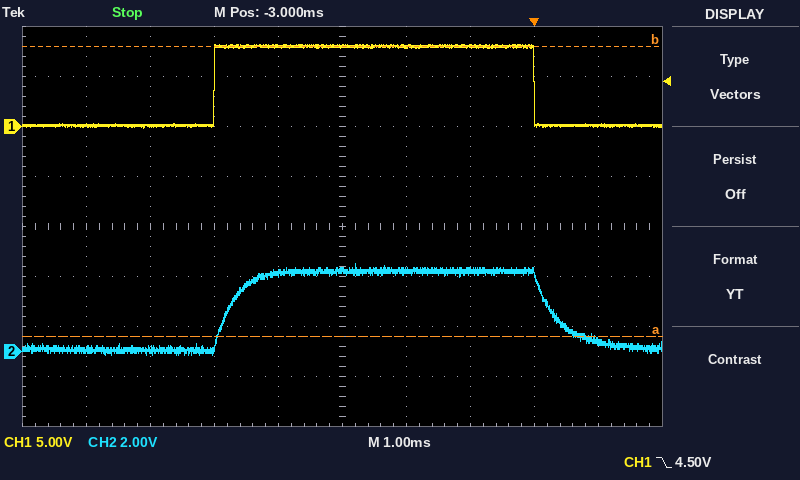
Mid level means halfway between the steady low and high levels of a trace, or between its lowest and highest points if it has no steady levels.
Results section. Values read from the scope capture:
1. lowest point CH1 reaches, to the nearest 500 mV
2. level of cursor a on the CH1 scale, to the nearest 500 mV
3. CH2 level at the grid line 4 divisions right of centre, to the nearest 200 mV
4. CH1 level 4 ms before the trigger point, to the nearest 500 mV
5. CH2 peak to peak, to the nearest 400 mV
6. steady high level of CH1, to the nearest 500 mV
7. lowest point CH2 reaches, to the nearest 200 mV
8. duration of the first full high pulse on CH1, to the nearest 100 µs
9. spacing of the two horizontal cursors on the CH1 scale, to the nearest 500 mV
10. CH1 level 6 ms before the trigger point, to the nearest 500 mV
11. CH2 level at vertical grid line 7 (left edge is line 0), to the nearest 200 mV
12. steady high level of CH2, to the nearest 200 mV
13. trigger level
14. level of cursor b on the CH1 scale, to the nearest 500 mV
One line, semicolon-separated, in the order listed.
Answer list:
0.0 V; -21.0 V; 400 mV; 8.0 V; 3.6 V; 8.0 V; -200 mV; 5.0 ms; 29.0 V; 0.0 V; 3.2 V; 3.2 V; 4.50 V; 8.0 V
